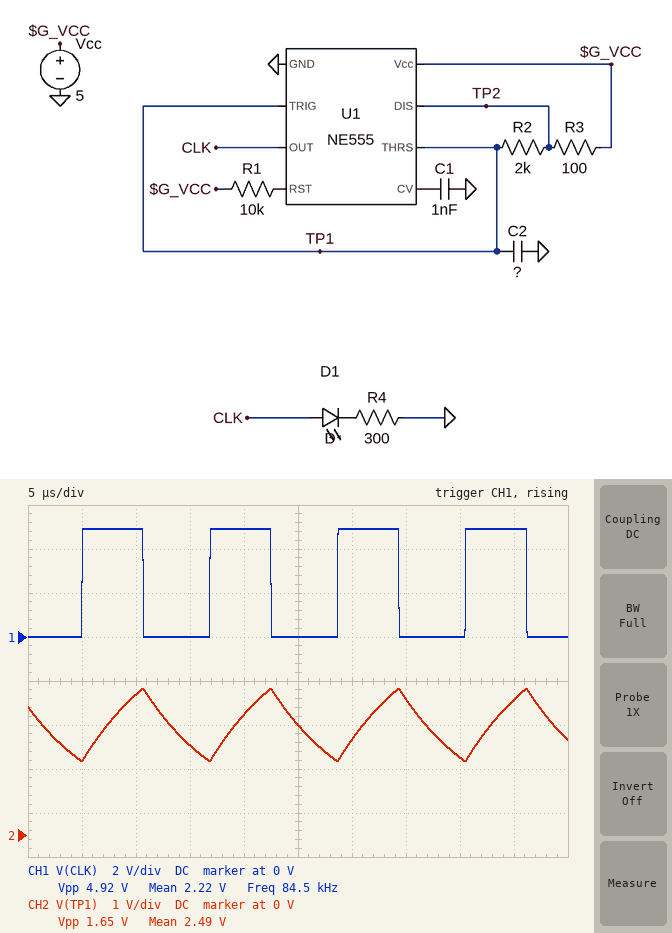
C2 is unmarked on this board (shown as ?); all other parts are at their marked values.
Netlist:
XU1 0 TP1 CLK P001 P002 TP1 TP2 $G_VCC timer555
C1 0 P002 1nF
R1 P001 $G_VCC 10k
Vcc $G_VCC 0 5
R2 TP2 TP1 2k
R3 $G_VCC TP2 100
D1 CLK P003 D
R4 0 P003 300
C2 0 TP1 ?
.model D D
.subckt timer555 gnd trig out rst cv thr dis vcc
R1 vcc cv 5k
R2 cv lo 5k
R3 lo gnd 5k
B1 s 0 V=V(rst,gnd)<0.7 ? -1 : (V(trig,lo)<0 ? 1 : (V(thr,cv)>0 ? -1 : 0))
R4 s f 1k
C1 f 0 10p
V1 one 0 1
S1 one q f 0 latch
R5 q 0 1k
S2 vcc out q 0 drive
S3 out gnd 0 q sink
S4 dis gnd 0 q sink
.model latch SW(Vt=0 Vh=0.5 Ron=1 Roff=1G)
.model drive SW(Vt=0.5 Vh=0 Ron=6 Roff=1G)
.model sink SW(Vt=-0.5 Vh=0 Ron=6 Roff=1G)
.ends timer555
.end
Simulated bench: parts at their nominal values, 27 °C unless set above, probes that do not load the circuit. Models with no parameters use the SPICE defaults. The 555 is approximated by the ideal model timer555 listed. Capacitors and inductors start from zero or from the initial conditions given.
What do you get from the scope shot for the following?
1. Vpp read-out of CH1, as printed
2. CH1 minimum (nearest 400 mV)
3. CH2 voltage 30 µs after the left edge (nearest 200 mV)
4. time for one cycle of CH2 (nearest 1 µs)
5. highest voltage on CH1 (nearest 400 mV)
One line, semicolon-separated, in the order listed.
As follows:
4.92 V; 0 V; 2.2 V; 12 µs; 4.8 V
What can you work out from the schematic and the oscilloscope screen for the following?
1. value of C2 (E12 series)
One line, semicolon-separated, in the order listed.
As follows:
3.9 nF
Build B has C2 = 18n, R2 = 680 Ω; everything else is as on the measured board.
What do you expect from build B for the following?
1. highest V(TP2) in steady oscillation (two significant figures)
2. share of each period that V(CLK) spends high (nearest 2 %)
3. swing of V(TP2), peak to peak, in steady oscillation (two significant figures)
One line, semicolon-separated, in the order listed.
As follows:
4.8 V; 50 %; 4.5 V
